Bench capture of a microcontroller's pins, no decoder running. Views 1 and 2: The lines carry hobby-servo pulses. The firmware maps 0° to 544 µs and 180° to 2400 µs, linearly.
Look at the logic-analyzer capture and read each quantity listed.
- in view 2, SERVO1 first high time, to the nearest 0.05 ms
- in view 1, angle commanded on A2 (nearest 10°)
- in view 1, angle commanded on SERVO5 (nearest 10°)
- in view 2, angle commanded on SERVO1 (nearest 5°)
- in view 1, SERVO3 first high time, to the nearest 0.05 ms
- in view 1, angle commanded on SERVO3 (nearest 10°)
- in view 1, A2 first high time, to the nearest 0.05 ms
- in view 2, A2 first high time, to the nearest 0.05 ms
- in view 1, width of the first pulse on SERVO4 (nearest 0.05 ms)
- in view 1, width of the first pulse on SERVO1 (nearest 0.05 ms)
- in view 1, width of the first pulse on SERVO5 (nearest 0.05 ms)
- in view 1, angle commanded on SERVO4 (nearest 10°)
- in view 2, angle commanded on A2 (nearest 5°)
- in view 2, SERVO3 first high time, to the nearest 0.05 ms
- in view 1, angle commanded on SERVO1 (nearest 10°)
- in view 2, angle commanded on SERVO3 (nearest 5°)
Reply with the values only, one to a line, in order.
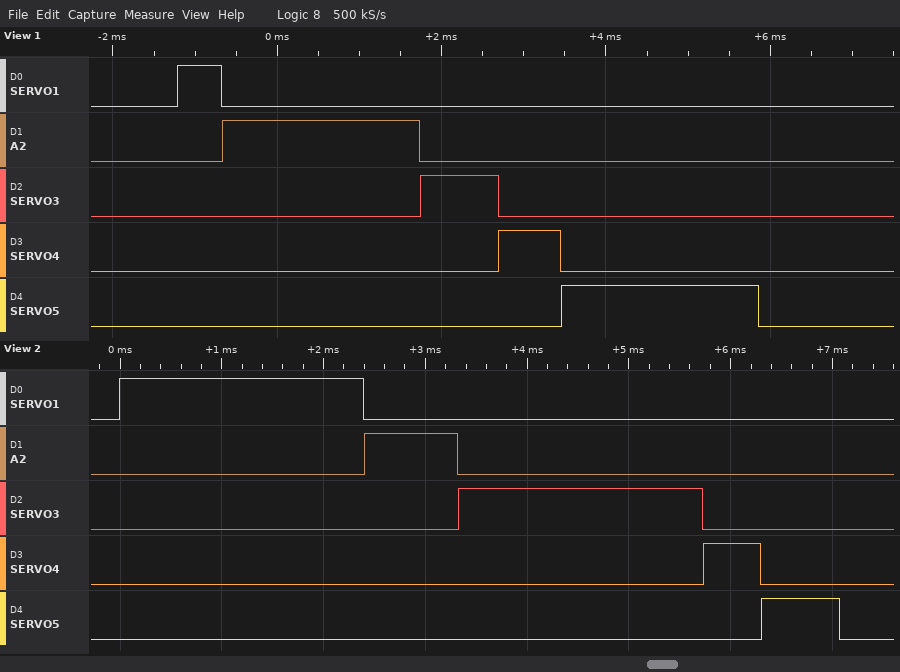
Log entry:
2.40 ms
180°
180°
180°
0.95 ms
40°
2.40 ms
0.90 ms
0.75 ms
0.55 ms
2.40 ms
20°
35°
2.40 ms
0°
180°
